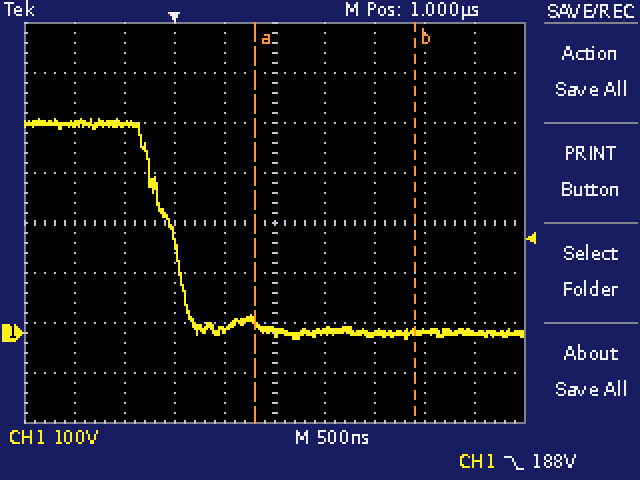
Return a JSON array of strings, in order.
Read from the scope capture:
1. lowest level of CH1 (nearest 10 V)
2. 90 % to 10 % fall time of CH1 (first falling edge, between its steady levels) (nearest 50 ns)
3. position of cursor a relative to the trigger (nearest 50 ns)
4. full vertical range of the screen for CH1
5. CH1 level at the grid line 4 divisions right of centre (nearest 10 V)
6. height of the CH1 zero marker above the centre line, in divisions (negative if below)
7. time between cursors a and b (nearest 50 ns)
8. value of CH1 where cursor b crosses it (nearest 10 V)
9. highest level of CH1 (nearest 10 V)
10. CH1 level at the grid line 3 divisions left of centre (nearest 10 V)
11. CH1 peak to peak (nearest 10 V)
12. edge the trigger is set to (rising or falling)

["-10 V", "450 ns", "+800 ns", "800 V", "0 V", "-2.2 div", "1.60 µs", "0 V", "430 V", "420 V", "440 V", "falling"]
